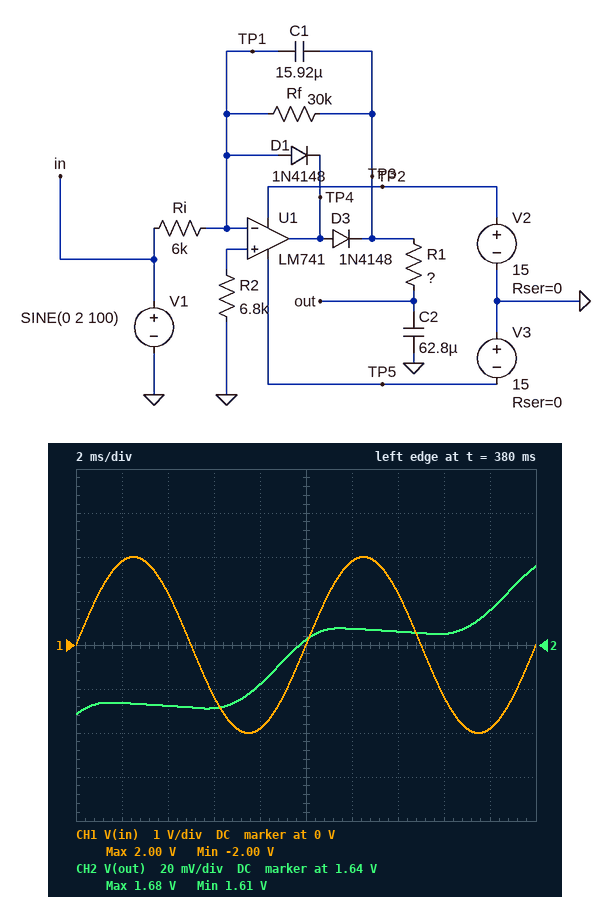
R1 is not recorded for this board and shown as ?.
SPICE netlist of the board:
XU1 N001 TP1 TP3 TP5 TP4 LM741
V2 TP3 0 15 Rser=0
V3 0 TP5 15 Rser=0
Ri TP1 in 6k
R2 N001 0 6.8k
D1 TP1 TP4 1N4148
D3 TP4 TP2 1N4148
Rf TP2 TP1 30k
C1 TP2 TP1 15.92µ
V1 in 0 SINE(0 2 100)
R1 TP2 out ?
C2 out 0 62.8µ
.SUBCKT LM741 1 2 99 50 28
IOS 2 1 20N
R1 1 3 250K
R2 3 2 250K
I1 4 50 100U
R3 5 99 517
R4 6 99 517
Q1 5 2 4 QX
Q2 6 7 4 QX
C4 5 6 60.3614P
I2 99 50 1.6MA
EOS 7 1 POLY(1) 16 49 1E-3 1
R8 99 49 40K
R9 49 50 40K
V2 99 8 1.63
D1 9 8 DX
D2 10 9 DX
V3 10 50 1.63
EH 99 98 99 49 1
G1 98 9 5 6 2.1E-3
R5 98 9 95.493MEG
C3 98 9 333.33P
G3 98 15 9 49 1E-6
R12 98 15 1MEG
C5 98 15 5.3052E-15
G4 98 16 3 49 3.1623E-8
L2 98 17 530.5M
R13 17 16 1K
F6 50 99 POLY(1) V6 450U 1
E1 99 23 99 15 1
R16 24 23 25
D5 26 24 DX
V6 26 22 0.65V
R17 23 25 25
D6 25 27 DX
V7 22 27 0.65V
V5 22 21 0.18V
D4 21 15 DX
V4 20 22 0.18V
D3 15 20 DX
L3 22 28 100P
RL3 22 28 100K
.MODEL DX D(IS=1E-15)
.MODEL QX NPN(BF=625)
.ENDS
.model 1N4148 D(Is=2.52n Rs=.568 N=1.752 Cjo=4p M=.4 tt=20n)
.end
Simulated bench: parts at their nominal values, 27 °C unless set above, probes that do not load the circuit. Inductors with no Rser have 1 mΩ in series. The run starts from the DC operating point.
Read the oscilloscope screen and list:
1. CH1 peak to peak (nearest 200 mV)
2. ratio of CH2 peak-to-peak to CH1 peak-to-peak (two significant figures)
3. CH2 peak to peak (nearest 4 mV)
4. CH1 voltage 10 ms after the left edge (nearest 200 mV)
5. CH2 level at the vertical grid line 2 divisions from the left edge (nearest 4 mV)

4.0 V
0.017
68 mV
0 V
1.612 V
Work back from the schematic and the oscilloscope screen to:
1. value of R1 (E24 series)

36 Ω
